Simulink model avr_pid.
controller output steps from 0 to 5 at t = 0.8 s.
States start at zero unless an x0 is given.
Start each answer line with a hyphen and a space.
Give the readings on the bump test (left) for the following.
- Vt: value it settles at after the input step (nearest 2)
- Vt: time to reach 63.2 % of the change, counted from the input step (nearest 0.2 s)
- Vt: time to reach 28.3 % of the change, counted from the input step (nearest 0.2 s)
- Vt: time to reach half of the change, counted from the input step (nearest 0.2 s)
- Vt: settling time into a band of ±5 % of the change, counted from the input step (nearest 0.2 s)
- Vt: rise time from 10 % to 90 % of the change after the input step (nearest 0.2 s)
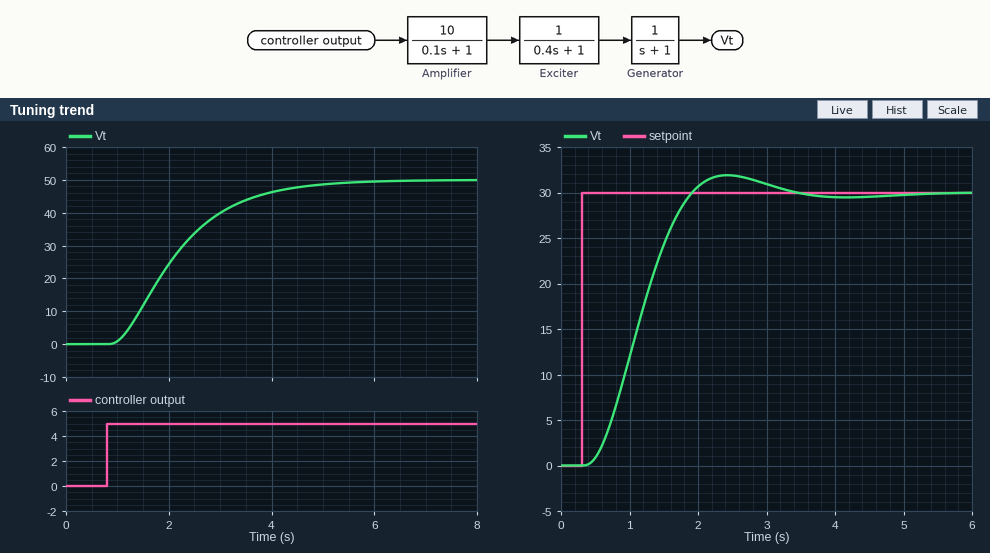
- 50
- 1.6 s
- 0.8 s
- 1.2 s
- 3.6 s
- 2.4 s
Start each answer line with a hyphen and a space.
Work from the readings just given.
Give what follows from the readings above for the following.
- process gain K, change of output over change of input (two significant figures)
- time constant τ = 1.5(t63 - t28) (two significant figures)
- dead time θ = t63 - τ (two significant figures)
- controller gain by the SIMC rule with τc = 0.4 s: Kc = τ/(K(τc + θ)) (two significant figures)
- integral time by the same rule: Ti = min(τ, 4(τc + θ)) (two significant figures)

- 10
- 1.2 s
- 0.40 s
- 0.15
- 1.2 s
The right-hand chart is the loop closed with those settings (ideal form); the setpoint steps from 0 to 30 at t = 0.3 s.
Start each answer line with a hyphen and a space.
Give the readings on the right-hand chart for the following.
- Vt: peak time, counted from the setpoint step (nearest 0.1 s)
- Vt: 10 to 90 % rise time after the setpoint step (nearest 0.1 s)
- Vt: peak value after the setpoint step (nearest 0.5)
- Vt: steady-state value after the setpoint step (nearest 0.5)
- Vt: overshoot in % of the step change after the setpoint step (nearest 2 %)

- 2.1 s
- 1.0 s
- 32.0
- 30.0
- 6 %
